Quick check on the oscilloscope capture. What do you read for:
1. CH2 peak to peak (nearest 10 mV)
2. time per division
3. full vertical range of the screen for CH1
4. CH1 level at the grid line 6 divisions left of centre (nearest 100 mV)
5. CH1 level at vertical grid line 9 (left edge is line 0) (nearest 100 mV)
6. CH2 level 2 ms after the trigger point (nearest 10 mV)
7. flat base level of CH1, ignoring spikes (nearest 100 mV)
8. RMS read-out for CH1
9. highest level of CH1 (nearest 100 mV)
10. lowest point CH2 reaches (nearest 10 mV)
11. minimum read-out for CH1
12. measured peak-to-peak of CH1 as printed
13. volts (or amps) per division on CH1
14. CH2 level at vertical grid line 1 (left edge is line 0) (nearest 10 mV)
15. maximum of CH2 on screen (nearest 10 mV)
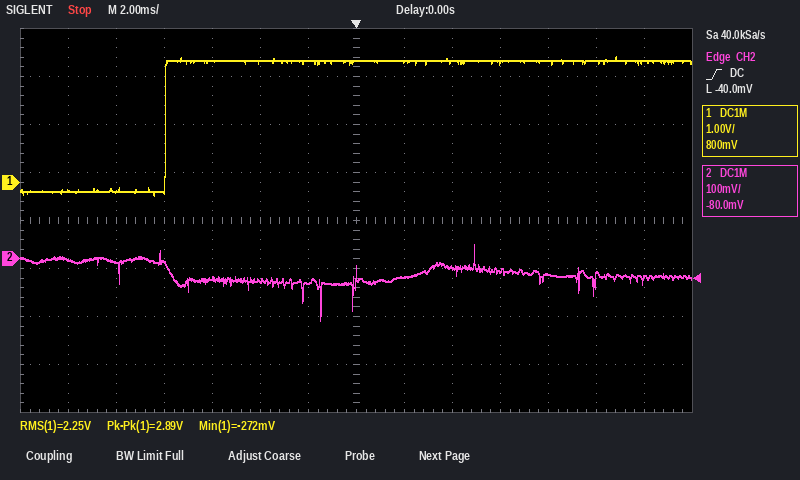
160 mV
2 ms
8 V
-200 mV
2.5 V
-40 mV
-200 mV
2.25 V
2.6 V
-130 mV
-272 mV
2.89 V
1 V
0 mV
30 mV
